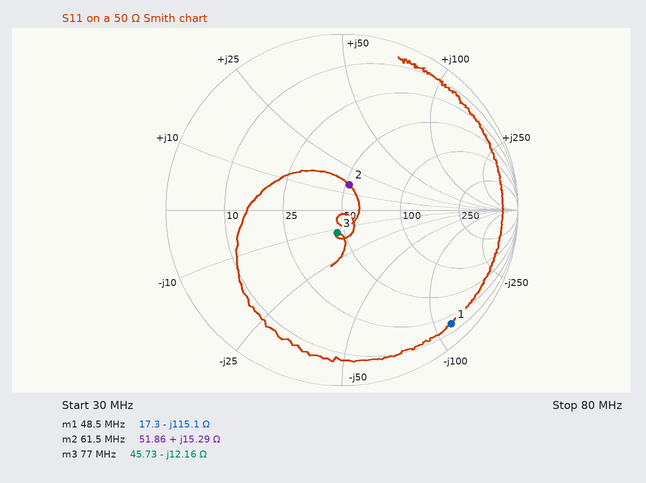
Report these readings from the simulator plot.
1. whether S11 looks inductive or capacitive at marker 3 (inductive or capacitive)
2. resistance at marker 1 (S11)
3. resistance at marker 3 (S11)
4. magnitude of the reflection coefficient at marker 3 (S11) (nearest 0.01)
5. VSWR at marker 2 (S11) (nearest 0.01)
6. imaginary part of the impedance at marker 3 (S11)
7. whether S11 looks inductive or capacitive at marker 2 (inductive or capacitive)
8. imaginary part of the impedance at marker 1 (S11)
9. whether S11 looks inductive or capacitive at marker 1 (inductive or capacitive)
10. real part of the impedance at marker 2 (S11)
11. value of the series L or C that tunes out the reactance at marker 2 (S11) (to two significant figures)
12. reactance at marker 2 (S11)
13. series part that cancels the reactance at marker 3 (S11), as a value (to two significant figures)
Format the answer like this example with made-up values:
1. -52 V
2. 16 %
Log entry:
1. capacitive
2. 17.3 Ω
3. 45.73 Ω
4. 0.13
5. 1.35
6. -12.16 Ω
7. inductive
8. -115.1 Ω
9. capacitive
10. 51.86 Ω
11. 170 pF
12. +15.29 Ω
13. 25 nH
